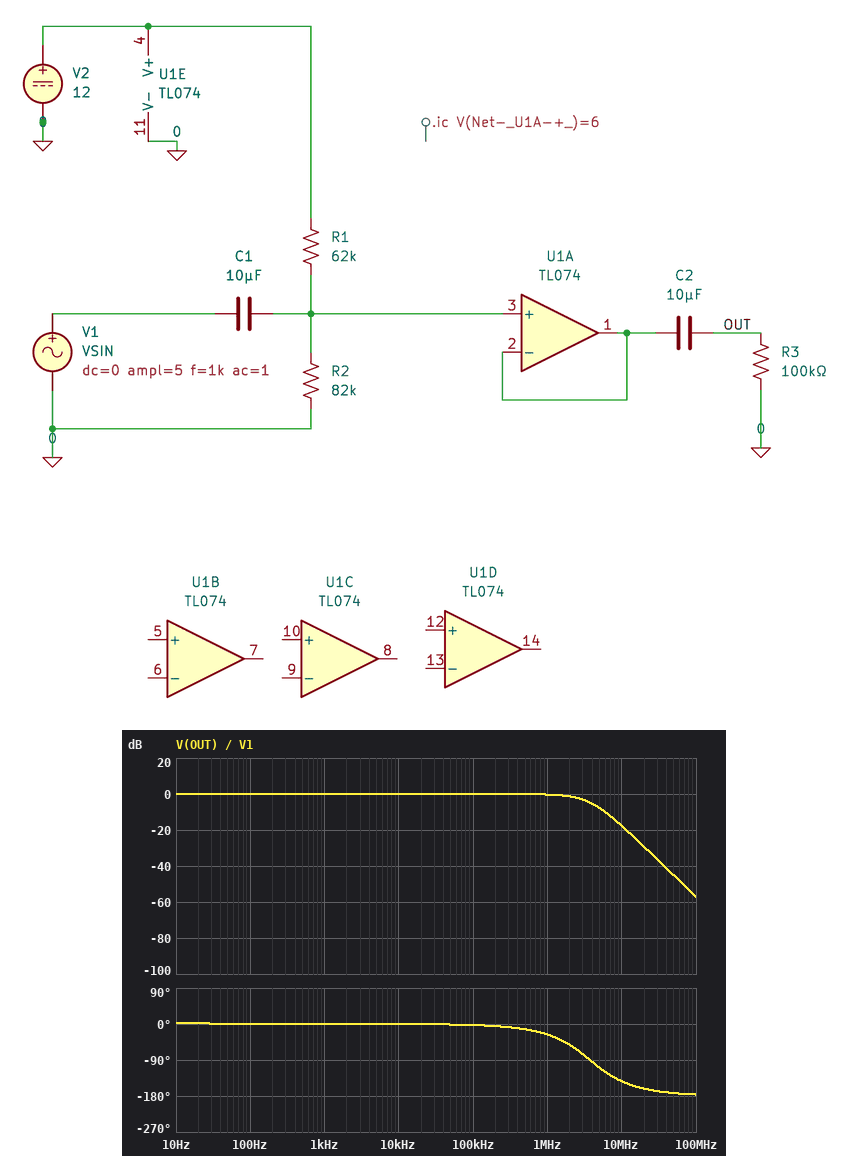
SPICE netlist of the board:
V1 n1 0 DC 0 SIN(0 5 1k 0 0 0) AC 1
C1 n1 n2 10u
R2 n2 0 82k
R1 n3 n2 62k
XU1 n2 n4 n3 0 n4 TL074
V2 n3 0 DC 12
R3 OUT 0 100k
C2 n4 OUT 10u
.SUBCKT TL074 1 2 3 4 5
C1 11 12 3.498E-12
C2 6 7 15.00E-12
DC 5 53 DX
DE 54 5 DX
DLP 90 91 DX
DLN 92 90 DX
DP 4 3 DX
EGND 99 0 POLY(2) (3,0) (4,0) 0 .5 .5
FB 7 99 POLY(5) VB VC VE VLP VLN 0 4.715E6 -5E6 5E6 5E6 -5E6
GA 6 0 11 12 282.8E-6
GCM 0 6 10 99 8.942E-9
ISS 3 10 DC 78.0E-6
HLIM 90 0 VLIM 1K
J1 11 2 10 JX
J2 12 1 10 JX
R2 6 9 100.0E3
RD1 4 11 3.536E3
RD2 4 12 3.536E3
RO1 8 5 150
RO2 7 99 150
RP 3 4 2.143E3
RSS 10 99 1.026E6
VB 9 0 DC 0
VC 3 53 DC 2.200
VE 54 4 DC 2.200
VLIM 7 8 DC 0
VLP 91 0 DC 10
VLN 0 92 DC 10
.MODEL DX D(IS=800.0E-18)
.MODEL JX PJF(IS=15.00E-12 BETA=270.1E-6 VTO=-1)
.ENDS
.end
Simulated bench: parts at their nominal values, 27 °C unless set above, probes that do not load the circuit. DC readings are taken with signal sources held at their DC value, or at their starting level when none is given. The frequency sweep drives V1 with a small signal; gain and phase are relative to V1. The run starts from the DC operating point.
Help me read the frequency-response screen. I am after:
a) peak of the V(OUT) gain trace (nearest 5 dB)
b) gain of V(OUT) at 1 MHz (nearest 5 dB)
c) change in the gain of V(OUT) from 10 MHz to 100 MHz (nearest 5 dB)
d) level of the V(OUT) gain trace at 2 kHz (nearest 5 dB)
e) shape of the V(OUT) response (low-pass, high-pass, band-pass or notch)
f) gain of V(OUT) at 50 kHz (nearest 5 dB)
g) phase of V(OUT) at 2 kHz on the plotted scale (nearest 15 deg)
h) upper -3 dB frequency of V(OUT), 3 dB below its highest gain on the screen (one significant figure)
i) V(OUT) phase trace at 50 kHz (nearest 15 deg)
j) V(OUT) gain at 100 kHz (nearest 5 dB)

0 dB
0 dB
-40 dB
0 dB
low-pass
0 dB
0 deg
3 MHz
0 deg
0 dB
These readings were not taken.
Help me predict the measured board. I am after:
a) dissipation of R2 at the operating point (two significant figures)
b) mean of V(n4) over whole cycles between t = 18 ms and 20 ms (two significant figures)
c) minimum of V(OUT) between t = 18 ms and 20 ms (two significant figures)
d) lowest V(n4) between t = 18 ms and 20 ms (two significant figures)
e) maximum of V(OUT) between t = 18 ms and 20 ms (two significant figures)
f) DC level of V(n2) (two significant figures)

570 µW
6.6 V
-5.0 V
1.8 V
3.6 V
6.8 V
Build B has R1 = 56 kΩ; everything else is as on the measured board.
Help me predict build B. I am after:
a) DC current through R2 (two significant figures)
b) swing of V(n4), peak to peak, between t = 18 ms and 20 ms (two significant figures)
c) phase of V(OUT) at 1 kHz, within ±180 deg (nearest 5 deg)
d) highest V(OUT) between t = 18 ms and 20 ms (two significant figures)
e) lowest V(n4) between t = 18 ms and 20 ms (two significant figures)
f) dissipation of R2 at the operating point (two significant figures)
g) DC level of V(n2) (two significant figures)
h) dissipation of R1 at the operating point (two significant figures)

87 µA
8.3 V
0 deg
3.3 V
2.1 V
620 µW
7.1 V
420 µW
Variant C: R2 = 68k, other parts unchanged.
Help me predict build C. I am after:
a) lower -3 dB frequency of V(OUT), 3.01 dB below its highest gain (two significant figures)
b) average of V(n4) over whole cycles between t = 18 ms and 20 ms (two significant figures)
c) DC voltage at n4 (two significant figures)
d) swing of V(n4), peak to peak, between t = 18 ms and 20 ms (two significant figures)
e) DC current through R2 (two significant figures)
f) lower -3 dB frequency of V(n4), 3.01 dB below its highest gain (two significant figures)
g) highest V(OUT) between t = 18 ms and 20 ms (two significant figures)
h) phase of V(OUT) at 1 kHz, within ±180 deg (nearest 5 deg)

540 mHz
6.2 V
6.3 V
8.9 V
92 µA
490 mHz
4.2 V
0 deg
